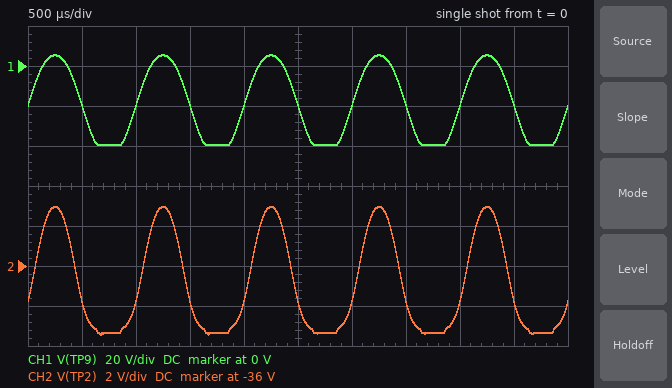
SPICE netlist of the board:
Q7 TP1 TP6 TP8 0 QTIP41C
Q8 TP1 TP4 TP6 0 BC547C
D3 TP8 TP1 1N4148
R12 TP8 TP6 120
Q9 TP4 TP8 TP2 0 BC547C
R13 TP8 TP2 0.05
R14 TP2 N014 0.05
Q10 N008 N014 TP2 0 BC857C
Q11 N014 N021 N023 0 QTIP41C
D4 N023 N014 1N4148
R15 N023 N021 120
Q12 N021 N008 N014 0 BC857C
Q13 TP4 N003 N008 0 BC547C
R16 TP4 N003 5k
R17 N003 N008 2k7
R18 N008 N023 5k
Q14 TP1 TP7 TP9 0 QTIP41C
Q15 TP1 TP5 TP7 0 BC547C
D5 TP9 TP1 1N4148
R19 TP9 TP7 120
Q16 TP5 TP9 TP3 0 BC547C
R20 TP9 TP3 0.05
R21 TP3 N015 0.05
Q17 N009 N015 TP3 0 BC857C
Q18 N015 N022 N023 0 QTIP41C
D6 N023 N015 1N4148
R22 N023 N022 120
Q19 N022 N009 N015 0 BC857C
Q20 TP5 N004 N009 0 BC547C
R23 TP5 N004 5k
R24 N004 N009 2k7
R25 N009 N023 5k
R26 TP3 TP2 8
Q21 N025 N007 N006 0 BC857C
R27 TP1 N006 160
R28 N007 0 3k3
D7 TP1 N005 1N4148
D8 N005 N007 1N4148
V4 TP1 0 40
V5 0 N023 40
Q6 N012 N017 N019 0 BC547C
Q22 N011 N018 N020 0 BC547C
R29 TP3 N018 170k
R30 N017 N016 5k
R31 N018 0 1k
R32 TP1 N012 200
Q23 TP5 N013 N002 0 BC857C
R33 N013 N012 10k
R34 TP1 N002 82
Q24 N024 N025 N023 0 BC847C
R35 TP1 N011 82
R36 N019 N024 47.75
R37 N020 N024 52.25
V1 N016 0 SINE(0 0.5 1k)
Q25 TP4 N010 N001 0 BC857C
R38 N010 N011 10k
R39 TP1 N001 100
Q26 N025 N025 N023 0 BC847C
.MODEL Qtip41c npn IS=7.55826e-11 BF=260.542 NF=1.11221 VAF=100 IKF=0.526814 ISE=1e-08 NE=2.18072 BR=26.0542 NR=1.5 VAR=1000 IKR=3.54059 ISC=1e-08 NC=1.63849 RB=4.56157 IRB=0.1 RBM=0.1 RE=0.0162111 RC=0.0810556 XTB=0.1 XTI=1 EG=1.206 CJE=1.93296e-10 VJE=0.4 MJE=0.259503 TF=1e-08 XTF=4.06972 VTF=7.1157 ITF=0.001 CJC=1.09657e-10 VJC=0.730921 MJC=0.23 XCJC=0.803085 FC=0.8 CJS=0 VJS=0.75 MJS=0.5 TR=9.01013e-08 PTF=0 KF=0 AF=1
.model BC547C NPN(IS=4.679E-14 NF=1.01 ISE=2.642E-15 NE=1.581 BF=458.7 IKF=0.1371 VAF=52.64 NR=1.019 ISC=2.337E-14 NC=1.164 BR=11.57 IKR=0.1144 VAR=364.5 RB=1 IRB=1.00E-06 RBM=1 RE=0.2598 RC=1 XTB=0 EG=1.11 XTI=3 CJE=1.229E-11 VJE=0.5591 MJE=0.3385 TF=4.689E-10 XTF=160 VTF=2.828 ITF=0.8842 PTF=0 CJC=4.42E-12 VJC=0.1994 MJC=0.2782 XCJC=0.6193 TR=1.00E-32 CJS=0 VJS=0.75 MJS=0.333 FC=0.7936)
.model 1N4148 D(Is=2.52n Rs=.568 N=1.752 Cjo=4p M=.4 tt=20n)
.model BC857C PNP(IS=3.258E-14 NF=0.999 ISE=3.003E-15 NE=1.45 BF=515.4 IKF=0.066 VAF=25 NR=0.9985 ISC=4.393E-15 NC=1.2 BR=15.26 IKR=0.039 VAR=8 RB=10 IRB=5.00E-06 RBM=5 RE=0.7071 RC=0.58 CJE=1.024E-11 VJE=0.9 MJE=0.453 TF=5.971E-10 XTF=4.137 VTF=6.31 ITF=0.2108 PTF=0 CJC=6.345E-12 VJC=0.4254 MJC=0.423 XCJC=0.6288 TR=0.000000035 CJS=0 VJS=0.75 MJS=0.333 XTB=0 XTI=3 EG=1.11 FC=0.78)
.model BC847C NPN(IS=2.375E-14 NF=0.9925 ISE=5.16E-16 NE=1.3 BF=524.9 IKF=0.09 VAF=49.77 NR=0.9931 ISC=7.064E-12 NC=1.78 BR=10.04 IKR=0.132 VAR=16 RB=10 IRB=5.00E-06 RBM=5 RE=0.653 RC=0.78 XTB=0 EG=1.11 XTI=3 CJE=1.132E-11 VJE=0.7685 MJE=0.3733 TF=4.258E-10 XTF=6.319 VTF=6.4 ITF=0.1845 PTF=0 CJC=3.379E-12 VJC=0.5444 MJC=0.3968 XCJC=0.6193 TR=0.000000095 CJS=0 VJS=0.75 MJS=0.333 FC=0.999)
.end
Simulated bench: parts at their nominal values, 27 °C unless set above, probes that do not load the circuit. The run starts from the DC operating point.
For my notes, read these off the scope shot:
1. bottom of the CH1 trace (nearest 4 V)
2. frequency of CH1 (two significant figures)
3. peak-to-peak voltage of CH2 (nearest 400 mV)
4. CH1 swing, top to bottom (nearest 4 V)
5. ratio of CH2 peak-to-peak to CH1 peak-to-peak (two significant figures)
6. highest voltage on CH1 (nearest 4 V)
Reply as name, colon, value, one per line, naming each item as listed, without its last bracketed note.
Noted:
bottom of the CH1 trace: -40 V
frequency of CH1: 1.0 kHz
peak-to-peak voltage of CH2: 6.4 V
CH1 swing, top to bottom: 44 V
ratio of CH2 peak-to-peak to CH1 peak-to-peak: 0.14
highest voltage on CH1: 4 V
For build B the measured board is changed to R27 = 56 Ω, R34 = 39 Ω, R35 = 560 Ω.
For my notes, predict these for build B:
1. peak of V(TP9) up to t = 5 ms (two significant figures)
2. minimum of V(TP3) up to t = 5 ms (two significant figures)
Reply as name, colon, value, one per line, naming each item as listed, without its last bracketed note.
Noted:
peak of V(TP9) up to t = 5 ms: 38 V
minimum of V(TP3) up to t = 5 ms: 4.6 V
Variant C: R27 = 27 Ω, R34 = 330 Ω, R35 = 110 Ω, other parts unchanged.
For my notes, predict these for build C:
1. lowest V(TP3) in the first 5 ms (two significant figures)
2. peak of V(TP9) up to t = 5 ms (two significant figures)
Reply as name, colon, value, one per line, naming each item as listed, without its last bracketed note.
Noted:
lowest V(TP3) in the first 5 ms: -5.6 V
peak of V(TP9) up to t = 5 ms: 15 V
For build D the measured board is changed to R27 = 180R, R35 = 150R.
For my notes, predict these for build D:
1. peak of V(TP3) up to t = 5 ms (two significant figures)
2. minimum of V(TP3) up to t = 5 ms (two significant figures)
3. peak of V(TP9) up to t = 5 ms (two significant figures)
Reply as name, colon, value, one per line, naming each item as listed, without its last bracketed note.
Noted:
peak of V(TP3) up to t = 5 ms: 870 mV
minimum of V(TP3) up to t = 5 ms: -39 V
peak of V(TP9) up to t = 5 ms: 1.1 V
